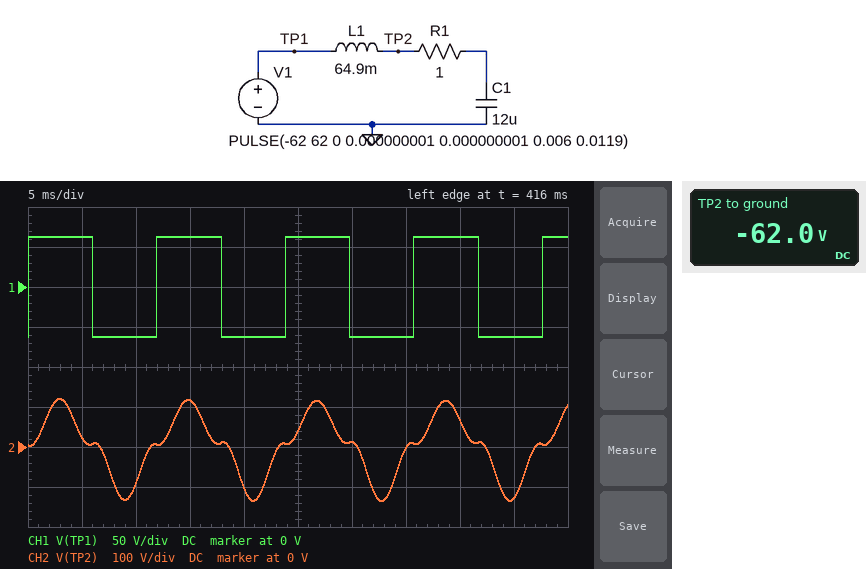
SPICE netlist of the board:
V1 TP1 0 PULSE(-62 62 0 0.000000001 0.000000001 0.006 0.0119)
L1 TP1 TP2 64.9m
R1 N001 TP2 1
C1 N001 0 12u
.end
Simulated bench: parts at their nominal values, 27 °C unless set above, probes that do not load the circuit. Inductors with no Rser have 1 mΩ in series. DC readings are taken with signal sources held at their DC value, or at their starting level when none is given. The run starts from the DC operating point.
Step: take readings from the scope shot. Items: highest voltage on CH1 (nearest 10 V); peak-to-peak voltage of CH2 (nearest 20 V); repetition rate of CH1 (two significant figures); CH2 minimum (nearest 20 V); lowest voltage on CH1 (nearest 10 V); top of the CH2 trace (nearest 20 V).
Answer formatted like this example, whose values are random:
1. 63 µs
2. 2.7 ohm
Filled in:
1. 60 V
2. 260 V
3. 84 Hz
4. -140 V
5. -60 V
6. 120 V
